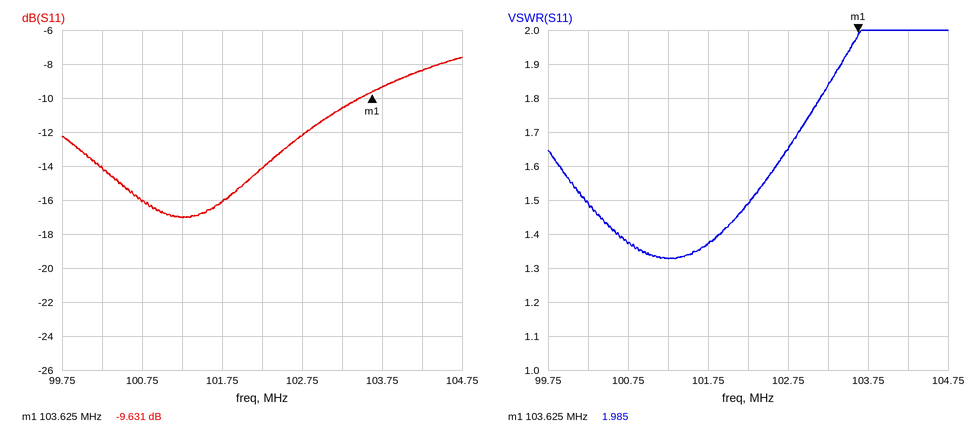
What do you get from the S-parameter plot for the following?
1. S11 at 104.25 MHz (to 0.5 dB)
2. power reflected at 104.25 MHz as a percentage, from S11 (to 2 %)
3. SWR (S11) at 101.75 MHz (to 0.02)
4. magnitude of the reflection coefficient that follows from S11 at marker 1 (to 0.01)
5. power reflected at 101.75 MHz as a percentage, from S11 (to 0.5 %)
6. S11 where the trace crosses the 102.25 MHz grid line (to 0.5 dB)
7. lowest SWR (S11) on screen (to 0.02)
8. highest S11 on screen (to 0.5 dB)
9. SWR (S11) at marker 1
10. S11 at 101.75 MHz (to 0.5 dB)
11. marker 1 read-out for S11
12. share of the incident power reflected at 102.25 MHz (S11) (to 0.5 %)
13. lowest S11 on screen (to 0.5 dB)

-8.5 dB
14 %
1.38
0.33
2.5 %
-14.0 dB
1.32
-7.5 dB
1.985
-16.0 dB
-9.631 dB
4.0 %
-17.0 dB
